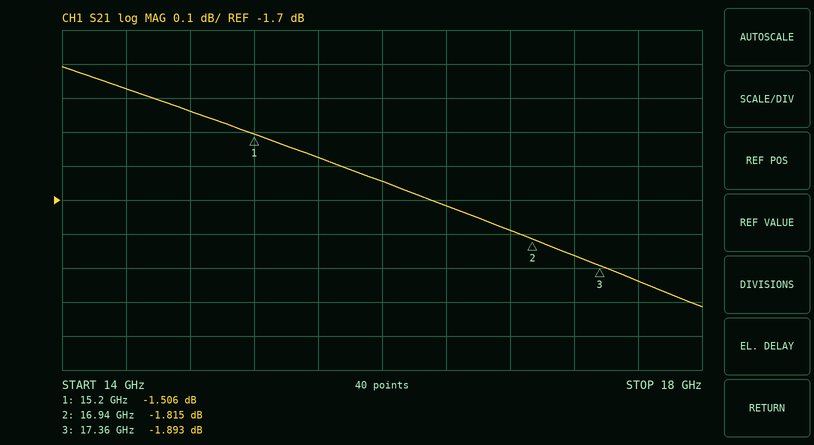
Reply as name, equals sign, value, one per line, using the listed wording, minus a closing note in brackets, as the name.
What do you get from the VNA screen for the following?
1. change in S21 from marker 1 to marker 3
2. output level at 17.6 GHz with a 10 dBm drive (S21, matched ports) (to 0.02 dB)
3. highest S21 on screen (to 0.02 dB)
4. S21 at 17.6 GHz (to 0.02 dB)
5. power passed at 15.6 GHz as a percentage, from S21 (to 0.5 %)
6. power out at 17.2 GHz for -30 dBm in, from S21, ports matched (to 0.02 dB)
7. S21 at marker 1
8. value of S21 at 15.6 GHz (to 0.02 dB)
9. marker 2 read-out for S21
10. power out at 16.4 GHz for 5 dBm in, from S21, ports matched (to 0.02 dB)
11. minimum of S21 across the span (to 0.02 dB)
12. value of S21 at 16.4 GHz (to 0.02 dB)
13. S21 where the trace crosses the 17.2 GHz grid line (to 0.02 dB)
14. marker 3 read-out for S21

change in S21 from marker 1 to marker 3 = -0.387 dB
output level at 17.6 GHz with a 10 dBm drive (S21, matched ports) = 8.06 dBm
highest S21 on screen = -1.30 dB
S21 at 17.6 GHz = -1.94 dB
power passed at 15.6 GHz as a percentage, from S21 = 69.5 %
power out at 17.2 GHz for -30 dBm in, from S21, ports matched = -31.86 dBm
S21 at marker 1 = -1.506 dB
value of S21 at 15.6 GHz = -1.58 dB
marker 2 read-out for S21 = -1.815 dB
power out at 16.4 GHz for 5 dBm in, from S21, ports matched = 3.28 dBm
minimum of S21 across the span = -2.02 dB
value of S21 at 16.4 GHz = -1.72 dB
S21 where the trace crosses the 17.2 GHz grid line = -1.86 dB
marker 3 read-out for S21 = -1.893 dB
